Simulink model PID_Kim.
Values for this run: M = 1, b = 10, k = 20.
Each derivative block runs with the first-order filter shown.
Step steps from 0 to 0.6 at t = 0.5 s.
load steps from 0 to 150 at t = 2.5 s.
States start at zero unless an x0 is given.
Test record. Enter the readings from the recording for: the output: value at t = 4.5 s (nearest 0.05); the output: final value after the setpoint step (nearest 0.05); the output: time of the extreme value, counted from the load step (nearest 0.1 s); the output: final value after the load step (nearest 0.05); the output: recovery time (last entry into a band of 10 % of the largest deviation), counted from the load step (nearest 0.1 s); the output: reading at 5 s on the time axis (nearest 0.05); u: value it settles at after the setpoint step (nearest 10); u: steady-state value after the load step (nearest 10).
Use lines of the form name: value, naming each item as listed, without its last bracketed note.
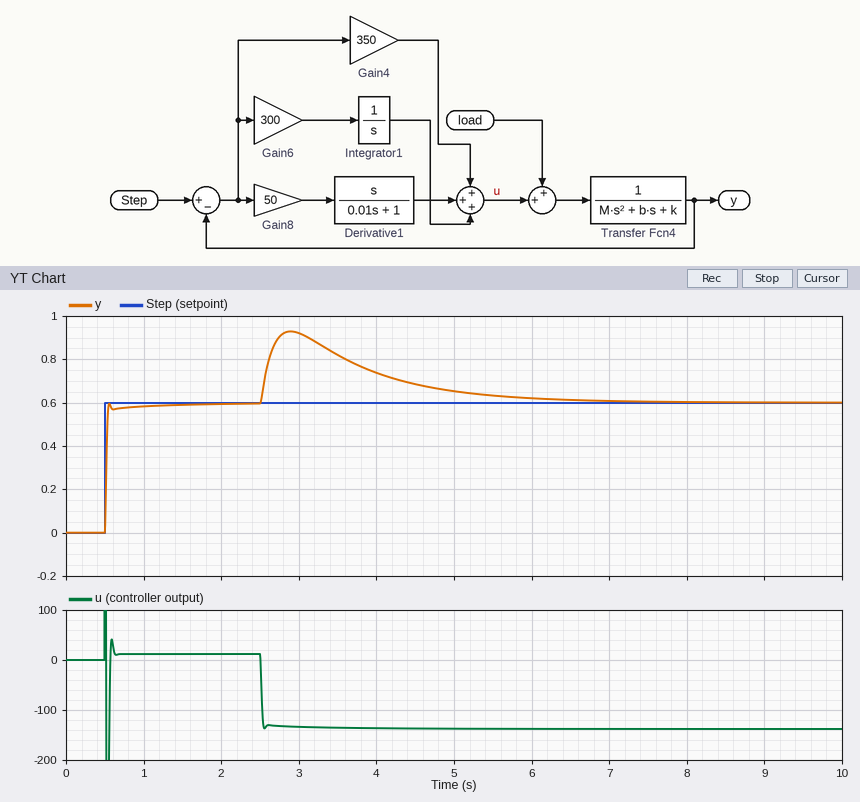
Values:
the output: value at t = 4.5 s: 0.70
the output: final value after the setpoint step: 0.60
the output: time of the extreme value, counted from the load step: 0.4 s
the output: final value after the load step: 0.60
the output: recovery time (last entry into a band of 10 % of the largest deviation), counted from the load step: 3.0 s
the output: reading at 5 s on the time axis: 0.65
u: value it settles at after the setpoint step: 10
u: steady-state value after the load step: -140
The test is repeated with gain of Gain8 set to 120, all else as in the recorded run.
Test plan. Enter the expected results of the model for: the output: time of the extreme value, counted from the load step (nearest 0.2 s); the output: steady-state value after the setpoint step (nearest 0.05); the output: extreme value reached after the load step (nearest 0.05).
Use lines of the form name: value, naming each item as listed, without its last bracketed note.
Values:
the output: time of the extreme value, counted from the load step: 0.6 s
the output: steady-state value after the setpoint step: 0.60
the output: extreme value reached after the load step: 0.90
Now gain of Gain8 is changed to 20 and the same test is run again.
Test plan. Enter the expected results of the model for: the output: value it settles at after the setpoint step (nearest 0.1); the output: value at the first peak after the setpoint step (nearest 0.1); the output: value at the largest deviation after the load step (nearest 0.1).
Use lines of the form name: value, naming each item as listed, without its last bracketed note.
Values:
the output: value it settles at after the setpoint step: 0.6
the output: value at the first peak after the setpoint step: 0.6
the output: value at the largest deviation after the load step: 1.0
